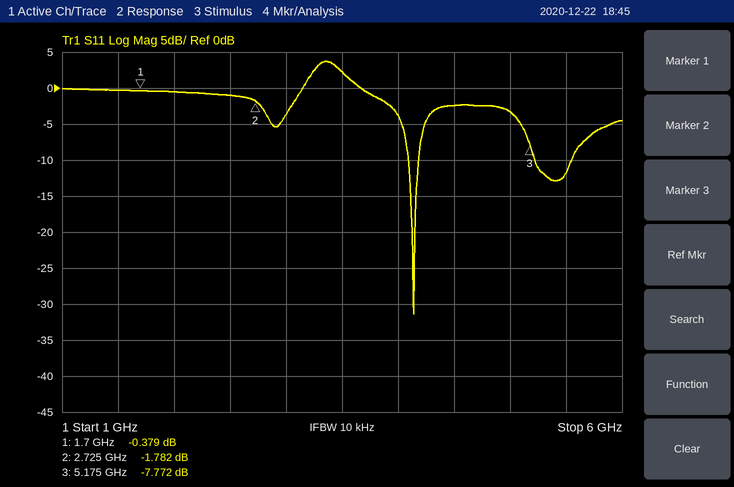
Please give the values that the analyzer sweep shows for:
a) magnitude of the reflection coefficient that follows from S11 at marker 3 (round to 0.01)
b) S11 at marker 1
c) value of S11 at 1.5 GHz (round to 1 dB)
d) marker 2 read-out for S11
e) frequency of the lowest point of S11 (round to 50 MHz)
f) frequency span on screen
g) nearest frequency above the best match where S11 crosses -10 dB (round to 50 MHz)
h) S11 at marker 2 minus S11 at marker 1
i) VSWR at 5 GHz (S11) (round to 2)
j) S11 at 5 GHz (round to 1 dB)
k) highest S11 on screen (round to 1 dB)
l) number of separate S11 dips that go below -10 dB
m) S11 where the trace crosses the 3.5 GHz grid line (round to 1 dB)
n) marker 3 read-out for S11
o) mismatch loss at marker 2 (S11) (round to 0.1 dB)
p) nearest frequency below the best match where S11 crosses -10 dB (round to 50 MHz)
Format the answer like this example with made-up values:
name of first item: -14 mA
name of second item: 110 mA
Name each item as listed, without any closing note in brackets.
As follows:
magnitude of the reflection coefficient that follows from S11 at marker 3: 0.41
S11 at marker 1: -0.379 dB
value of S11 at 1.5 GHz: 0 dB
marker 2 read-out for S11: -1.782 dB
frequency of the lowest point of S11: 4.15 GHz
frequency span on screen: 5 GHz
nearest frequency above the best match where S11 crosses -10 dB: 4.20 GHz
S11 at marker 2 minus S11 at marker 1: -1.403 dB
VSWR at 5 GHz (S11): 6
S11 at 5 GHz: -3 dB
highest S11 on screen: 4 dB
number of separate S11 dips that go below -10 dB: 2
S11 where the trace crosses the 3.5 GHz grid line: 2 dB
marker 3 read-out for S11: -7.772 dB
mismatch loss at marker 2 (S11): 4.7 dB
nearest frequency below the best match where S11 crosses -10 dB: 4.10 GHz
